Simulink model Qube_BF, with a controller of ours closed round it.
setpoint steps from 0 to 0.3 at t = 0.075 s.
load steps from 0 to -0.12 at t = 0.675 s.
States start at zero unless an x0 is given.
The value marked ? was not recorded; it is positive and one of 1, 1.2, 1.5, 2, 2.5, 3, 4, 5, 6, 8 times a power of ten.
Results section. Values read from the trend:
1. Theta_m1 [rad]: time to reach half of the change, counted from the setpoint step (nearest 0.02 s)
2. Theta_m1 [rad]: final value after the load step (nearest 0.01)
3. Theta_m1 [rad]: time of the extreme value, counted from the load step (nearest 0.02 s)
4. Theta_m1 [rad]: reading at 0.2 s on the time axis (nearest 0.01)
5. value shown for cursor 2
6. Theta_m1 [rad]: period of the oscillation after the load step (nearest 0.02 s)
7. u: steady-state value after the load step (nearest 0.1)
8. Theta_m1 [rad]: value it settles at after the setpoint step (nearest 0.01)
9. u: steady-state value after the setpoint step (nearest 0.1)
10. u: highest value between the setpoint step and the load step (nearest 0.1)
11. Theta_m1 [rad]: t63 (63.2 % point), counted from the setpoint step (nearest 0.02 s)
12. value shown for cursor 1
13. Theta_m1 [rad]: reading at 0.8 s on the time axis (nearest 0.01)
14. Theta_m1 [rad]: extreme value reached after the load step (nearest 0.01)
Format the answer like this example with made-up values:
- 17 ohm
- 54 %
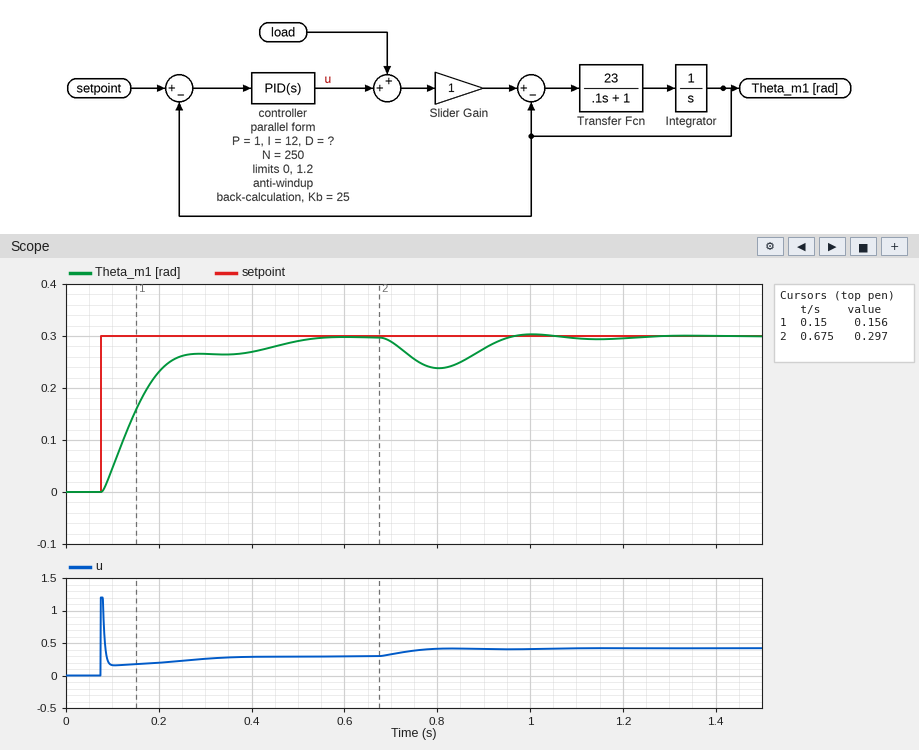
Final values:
- 0.08 s
- 0.30
- 0.12 s
- 0.23
- 0.297
- 0.34 s
- 0.4
- 0.30
- 0.3
- 1.2
- 0.10 s
- 0.156
- 0.24
- 0.24
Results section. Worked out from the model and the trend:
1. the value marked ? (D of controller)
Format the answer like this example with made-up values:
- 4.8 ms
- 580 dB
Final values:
- 0.04
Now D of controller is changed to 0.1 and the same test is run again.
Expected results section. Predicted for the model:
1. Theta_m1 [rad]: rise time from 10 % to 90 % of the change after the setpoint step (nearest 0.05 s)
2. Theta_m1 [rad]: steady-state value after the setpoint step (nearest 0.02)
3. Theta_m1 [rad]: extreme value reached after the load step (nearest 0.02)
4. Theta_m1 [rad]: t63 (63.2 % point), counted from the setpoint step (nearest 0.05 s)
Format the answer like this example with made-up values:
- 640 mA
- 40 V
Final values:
- 0.30 s
- 0.30
- 0.26
- 0.20 s
